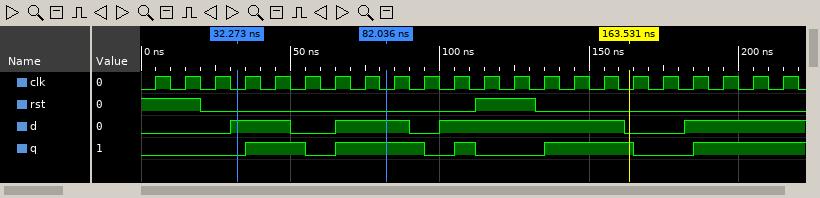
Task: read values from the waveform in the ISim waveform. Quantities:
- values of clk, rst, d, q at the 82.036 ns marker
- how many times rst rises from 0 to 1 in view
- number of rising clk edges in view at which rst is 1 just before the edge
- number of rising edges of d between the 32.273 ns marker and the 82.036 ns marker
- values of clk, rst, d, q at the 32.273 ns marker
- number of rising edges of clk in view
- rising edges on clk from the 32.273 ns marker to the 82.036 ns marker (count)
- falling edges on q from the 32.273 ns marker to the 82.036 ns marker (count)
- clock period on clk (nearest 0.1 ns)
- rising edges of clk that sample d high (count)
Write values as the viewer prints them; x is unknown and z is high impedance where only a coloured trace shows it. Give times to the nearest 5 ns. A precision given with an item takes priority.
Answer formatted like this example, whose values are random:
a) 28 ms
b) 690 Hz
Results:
a) clk=0, rst=0, d=1, q=1
b) 1
c) 4
d) 1
e) clk=0, rst=0, d=1, q=0
f) 22
g) 5
h) 1
i) 10 ns
j) 14
